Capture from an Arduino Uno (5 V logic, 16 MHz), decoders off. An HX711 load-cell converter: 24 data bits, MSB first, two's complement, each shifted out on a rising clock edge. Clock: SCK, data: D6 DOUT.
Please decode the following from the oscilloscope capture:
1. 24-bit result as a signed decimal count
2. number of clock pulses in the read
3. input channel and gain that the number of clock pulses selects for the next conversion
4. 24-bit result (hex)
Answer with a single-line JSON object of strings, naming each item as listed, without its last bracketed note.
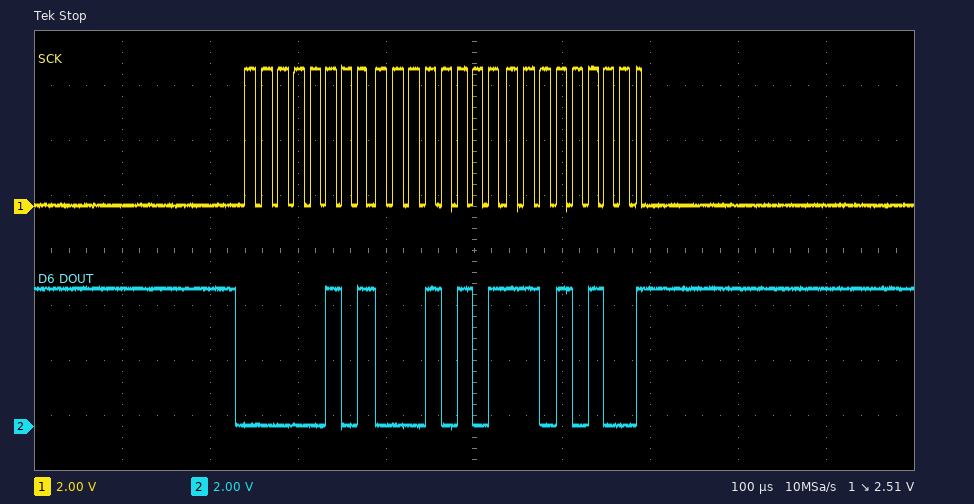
{"24-bit result as a signed decimal count": "333268", "number of clock pulses in the read": "25", "input channel and gain that the number of clock pulses selects for the next conversion": "channel A, gain 128", "24-bit result": "0x0515D4"}
